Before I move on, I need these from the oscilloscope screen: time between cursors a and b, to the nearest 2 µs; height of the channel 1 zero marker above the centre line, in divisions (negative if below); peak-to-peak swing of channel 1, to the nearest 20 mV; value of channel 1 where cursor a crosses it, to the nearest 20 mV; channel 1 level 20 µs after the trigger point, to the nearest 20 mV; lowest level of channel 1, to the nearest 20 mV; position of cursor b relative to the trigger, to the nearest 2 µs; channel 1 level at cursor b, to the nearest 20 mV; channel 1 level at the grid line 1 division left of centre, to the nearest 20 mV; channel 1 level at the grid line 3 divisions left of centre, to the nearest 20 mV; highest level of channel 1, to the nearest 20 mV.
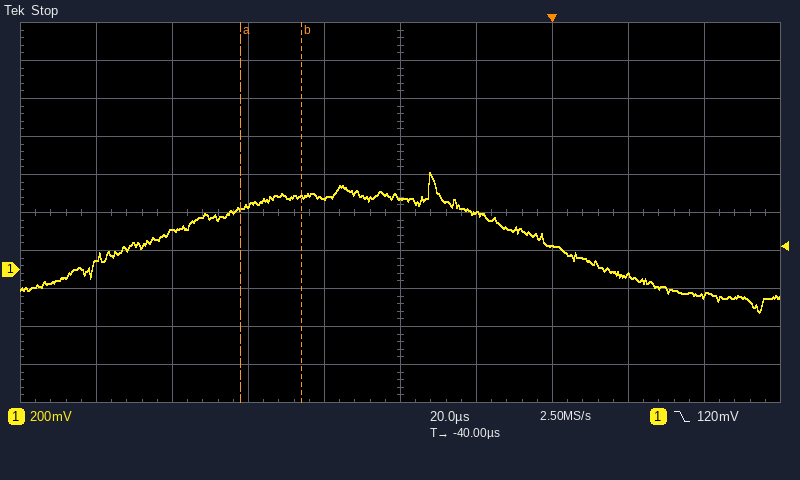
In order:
16 µs
-1.5 div
740 mV
320 mV
-40 mV
-220 mV
-66 µs
380 mV
380 mV
200 mV
520 mV
